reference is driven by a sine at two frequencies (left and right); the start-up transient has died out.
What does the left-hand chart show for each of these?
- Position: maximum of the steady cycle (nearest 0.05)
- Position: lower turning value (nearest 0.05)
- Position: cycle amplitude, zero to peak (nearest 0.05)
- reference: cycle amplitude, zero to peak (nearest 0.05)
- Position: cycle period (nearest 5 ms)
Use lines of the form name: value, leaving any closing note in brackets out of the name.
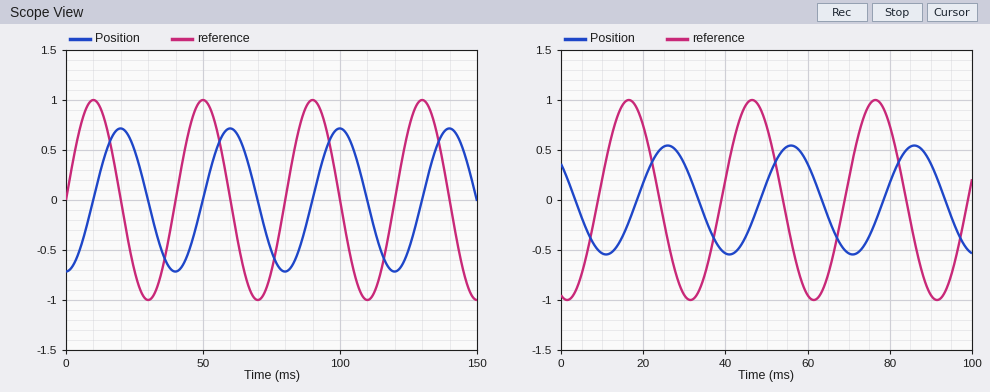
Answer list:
Position: maximum of the steady cycle: 0.70
Position: lower turning value: -0.70
Position: cycle amplitude, zero to peak: 0.70
reference: cycle amplitude, zero to peak: 1.00
Position: cycle period: 40 ms
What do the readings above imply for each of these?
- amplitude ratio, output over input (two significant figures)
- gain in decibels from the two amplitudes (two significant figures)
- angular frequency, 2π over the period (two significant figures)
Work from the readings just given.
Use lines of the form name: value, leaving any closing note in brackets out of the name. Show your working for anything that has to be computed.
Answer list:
amplitude ratio, output over input: 0.7 / 1 = 0.70
gain in decibels from the two amplitudes: 20 log10(0.7 / 1) = -3.1 dB
angular frequency, 2π over the period: 2π / 40 = 0.16 rad/ms
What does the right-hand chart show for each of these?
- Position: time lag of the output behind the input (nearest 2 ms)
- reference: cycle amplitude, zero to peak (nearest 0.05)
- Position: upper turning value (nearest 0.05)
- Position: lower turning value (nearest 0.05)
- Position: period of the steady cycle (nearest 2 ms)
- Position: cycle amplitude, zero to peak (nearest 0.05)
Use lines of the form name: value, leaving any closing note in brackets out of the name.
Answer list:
Position: time lag of the output behind the input: 10 ms
reference: cycle amplitude, zero to peak: 1.00
Position: upper turning value: 0.55
Position: lower turning value: -0.55
Position: period of the steady cycle: 30 ms
Position: cycle amplitude, zero to peak: 0.55
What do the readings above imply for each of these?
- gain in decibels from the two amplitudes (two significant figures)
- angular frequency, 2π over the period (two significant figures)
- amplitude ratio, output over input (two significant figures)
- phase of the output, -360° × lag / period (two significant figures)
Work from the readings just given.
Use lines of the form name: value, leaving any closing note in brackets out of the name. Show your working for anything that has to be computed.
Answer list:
gain in decibels from the two amplitudes: 20 log10(0.55 / 1) = -5.2 dB
angular frequency, 2π over the period: 2π / 30 = 0.21 rad/ms
amplitude ratio, output over input: 0.55 / 1 = 0.55
phase of the output, -360° × lag / period: -360 × 10 / 30 = -120°
